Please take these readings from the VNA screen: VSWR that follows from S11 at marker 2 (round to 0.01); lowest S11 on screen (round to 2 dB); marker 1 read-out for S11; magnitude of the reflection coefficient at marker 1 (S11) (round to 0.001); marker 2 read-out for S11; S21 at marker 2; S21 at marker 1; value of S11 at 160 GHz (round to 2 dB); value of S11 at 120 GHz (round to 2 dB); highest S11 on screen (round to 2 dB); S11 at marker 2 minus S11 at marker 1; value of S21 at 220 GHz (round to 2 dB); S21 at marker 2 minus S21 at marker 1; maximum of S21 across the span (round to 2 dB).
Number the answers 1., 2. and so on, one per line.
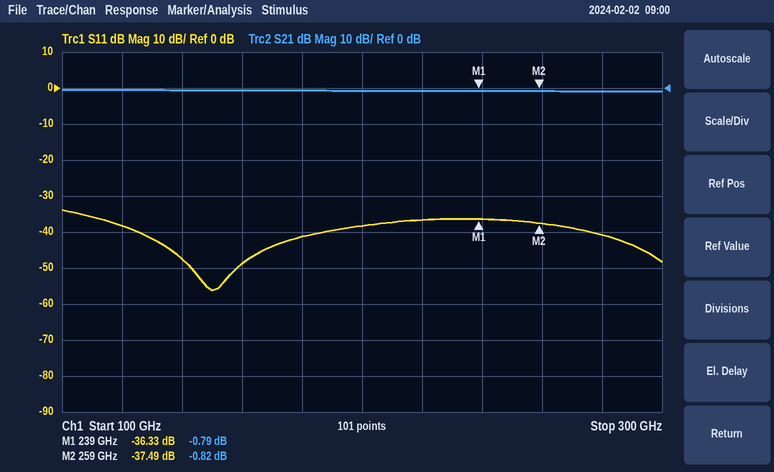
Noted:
1. 1.03
2. -56 dB
3. -36.33 dB
4. 0.015
5. -37.49 dB
6. -0.82 dB
7. -0.79 dB
8. -48 dB
9. -38 dB
10. -34 dB
11. -1.16 dB
12. 0 dB
13. -0.03 dB
14. 0 dB
